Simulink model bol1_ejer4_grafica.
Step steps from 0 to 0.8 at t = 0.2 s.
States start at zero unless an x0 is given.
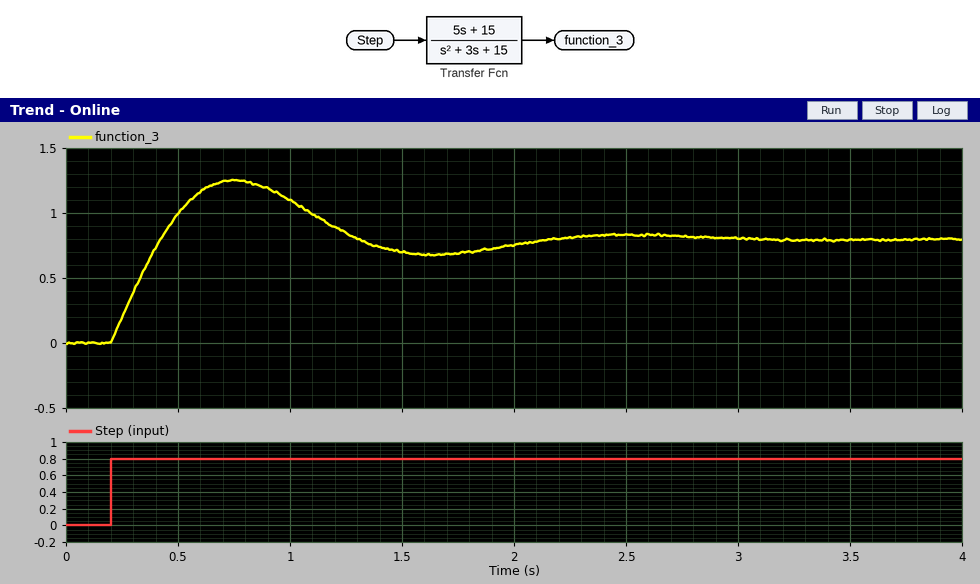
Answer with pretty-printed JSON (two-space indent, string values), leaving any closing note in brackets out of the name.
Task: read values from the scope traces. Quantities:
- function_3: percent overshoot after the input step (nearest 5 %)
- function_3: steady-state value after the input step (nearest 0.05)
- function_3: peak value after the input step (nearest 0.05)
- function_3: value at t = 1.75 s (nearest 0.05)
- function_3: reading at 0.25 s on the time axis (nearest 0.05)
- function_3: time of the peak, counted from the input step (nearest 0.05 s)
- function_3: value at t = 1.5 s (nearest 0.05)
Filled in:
{
  "function_3: percent overshoot after the input step": "55 %",
  "function_3: steady-state value after the input step": "0.80",
  "function_3: peak value after the input step": "1.25",
  "function_3: value at t = 1.75 s": "0.70",
  "function_3: reading at 0.25 s on the time axis": "0.20",
  "function_3: time of the peak, counted from the input step": "0.55 s",
  "function_3: value at t = 1.5 s": "0.70"
}
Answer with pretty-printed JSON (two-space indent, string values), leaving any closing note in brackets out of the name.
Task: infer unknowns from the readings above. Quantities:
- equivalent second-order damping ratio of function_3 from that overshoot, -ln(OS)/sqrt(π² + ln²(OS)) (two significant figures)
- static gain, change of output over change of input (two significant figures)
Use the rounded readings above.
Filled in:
{
  "equivalent second-order damping ratio of function_3 from that overshoot, -ln(OS)/sqrt(π² + ln²(OS))": "0.19",
  "static gain, change of output over change of input": "1.0"
}
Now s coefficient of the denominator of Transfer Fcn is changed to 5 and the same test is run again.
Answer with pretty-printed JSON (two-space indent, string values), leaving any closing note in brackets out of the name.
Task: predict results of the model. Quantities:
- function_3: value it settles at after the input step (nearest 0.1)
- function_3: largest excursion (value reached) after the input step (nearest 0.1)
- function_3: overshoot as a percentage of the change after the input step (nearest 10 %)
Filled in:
{
  "function_3: value it settles at after the input step": "0.8",
  "function_3: largest excursion (value reached) after the input step": "1.0",
  "function_3: overshoot as a percentage of the change after the input step": "20 %"
}
